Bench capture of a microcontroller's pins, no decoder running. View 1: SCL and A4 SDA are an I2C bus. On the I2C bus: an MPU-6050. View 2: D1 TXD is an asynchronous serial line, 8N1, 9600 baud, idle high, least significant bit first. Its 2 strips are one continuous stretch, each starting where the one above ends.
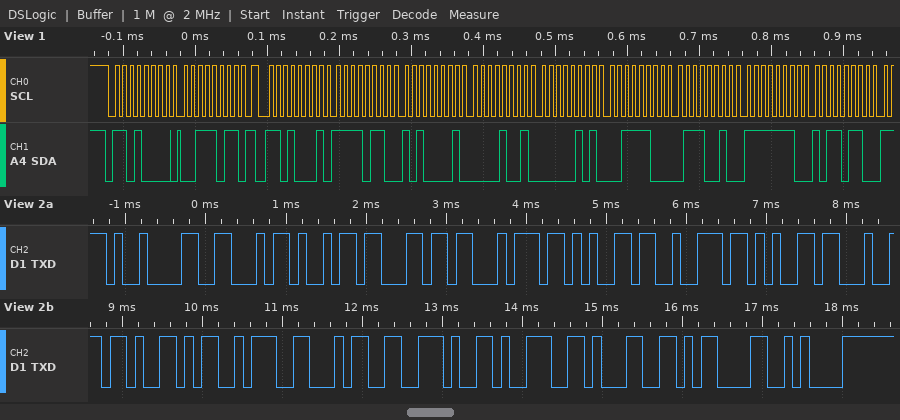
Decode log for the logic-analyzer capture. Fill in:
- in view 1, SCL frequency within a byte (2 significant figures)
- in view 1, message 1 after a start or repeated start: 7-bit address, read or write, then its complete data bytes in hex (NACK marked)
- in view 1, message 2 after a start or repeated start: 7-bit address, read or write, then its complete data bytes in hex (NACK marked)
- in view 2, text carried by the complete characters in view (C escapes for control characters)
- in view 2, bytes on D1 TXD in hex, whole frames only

100 kHz
0x68 write: 3B
0x68 read: F6 A1 09 05 3C 72 FE B6
"\tFilteredY:4.91\r\n"
0x09 0x46 0x69 0x6C 0x74 0x65 0x72 0x65 0x64 0x59 0x3A 0x34 0x2E 0x39 0x31 0x0D 0x0A
